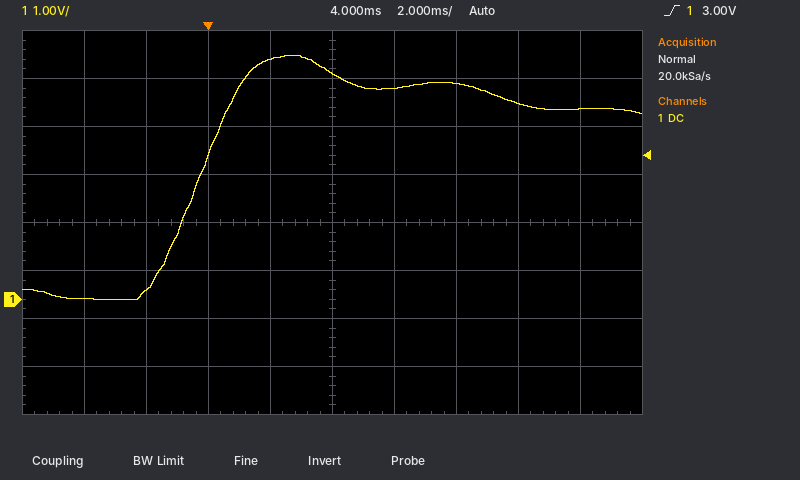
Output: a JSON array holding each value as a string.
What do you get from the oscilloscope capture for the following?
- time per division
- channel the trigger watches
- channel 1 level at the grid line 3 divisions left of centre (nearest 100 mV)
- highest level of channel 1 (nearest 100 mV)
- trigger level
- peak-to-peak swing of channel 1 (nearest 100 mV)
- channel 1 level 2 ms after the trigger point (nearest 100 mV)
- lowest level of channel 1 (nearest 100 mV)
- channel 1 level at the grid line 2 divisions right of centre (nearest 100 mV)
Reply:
["2 ms", "channel 1", "200 mV", "5.1 V", "3.00 V", "5.1 V", "5.0 V", "0.0 V", "4.5 V"]
